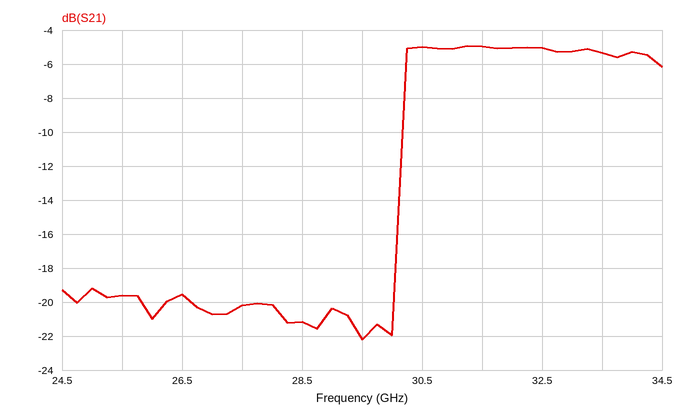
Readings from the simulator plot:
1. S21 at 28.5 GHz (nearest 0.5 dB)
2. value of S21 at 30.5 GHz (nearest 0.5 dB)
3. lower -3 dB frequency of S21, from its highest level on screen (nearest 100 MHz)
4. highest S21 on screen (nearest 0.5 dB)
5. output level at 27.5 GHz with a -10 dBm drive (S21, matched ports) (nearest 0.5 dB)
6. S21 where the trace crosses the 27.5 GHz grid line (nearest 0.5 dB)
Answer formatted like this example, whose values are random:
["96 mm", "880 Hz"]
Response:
["-21.0 dB", "-5.0 dB", "30.2 GHz", "-5.0 dB", "-30.0 dBm", "-20.0 dB"]
